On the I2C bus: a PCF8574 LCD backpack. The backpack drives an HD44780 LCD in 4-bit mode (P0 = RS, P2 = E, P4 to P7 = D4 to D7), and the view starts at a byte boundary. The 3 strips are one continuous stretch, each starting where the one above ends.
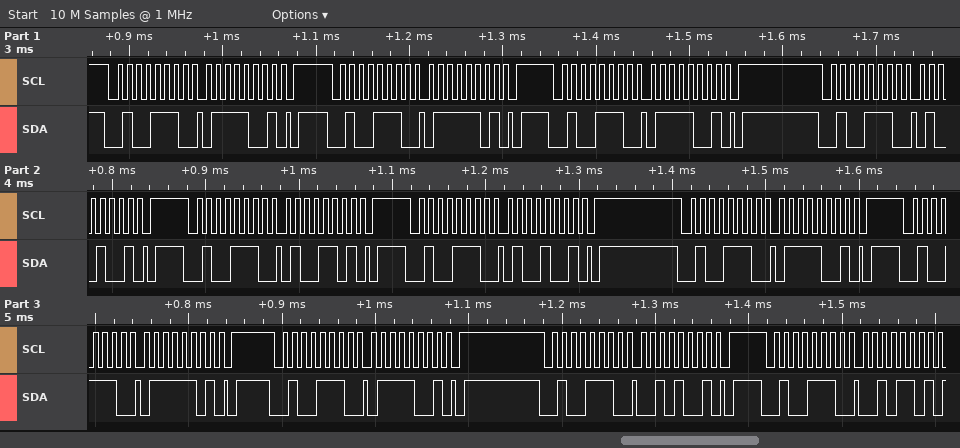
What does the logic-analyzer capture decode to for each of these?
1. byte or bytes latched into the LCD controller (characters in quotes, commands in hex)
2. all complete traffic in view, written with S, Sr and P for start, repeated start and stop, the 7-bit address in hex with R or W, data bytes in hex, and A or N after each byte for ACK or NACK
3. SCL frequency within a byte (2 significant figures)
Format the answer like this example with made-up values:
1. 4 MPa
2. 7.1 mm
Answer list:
1. 't'
2. S 27W A 79 A P S 27W A 7D A P S 27W A 79 A P S 27W A 49 A P S 27W A 4D A P S 27W A 49 A P S 27W A 79 A P S 27W A 7D A P S 27W A 79 A P S 27W A 29 A P S 27W A 2D A
3. 100 kHz
